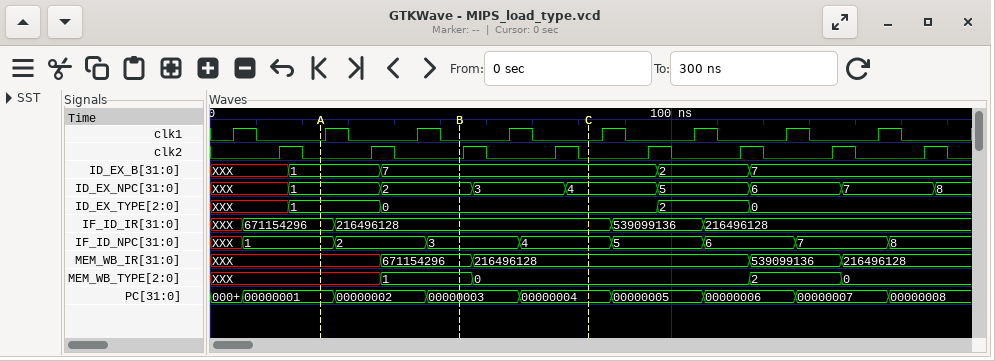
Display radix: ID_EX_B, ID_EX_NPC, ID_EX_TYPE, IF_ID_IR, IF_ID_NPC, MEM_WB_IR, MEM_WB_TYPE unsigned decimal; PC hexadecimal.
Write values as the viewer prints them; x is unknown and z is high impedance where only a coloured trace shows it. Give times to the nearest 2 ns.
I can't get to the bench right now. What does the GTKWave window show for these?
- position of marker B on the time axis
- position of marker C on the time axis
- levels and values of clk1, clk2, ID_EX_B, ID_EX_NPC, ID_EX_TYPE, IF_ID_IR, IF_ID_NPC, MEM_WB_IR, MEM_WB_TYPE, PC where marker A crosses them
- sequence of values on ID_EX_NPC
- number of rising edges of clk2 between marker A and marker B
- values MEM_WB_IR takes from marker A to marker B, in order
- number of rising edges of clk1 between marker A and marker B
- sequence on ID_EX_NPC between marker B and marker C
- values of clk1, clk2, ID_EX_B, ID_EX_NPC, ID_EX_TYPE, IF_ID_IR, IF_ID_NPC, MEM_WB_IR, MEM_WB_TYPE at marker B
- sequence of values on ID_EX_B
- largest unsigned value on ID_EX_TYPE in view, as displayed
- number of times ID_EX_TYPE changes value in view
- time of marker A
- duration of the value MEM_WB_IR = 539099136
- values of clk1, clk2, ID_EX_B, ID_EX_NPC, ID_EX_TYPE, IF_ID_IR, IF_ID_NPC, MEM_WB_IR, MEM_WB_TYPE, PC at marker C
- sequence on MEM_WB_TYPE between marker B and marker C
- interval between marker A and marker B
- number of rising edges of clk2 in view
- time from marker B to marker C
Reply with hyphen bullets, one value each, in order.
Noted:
- 54 ns
- 82 ns
- clk1=0, clk2=0, ID_EX_B=1, ID_EX_NPC=1, ID_EX_TYPE=1, IF_ID_IR=671154296, IF_ID_NPC=1, MEM_WB_IR=XXX, MEM_WB_TYPE=XXX, PC=00000001
- XXX, 1, 2, 3, 4, 5, 6, 7, 8
- 1
- XXX, 671154296
- 2
- 2, 3, 4
- clk1=0, clk2=0, ID_EX_B=7, ID_EX_NPC=2, ID_EX_TYPE=0, IF_ID_IR=216496128, IF_ID_NPC=3, MEM_WB_IR=671154296, MEM_WB_TYPE=1
- XXX, 1, 7, 2, 7
- 2
- 4
- 24 ns
- 20 ns
- clk1=0, clk2=0, ID_EX_B=7, ID_EX_NPC=4, ID_EX_TYPE=0, IF_ID_IR=216496128, IF_ID_NPC=4, MEM_WB_IR=216496128, MEM_WB_TYPE=0, PC=00000004
- 1, 0
- 30 ns
- 8
- 28 ns
